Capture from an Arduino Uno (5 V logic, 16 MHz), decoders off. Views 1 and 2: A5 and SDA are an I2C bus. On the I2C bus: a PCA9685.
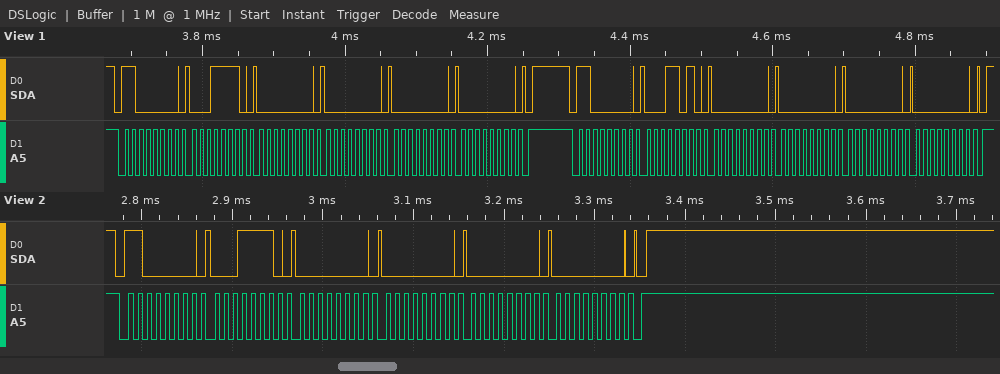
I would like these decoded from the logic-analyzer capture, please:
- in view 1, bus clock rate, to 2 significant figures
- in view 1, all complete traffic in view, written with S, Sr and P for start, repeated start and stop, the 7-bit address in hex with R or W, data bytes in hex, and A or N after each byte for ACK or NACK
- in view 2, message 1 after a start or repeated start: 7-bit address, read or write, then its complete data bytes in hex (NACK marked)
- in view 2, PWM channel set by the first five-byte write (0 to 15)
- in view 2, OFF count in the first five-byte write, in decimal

100 kHz
S 60W A 1E A 00 A 00 A 00 A 00 A P S 60W A 1A A 00 A 00 A 00 A 00 A P
0x60 write: 1E 00 00 00 00
6
0
